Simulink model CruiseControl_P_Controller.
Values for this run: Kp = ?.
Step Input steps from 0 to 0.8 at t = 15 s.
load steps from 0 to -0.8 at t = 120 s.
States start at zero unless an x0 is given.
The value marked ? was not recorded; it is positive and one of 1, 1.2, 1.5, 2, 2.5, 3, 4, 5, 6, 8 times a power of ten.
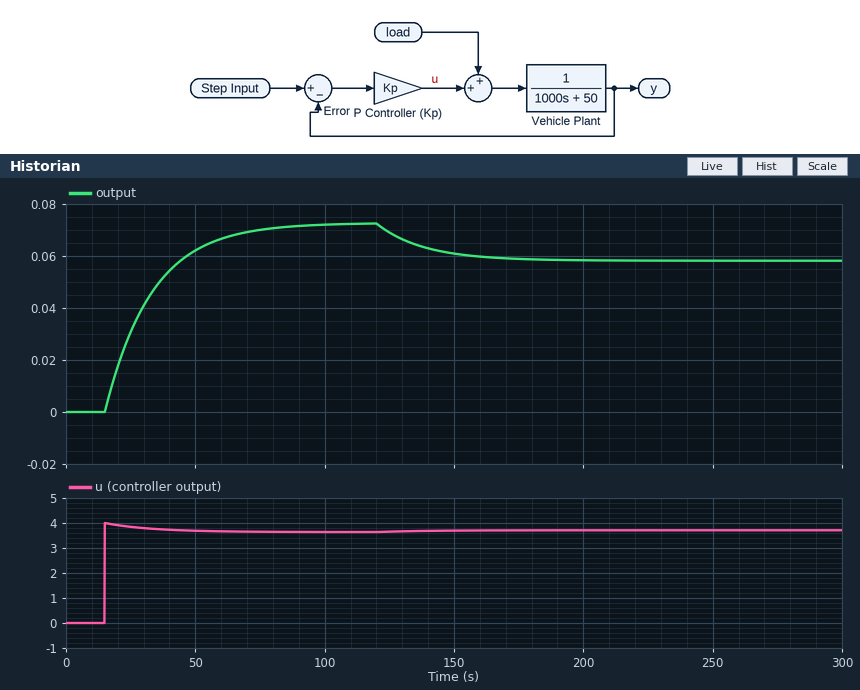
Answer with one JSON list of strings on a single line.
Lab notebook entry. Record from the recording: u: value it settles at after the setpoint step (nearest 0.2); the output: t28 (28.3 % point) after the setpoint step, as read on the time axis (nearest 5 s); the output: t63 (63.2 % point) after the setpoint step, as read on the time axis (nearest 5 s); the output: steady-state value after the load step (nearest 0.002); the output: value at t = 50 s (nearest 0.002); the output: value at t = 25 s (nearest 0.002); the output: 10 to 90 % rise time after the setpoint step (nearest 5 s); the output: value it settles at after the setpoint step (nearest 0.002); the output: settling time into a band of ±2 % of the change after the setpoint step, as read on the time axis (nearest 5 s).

["3.6", "20 s", "35 s", "0.058", "0.062", "0.030", "40 s", "0.072", "85 s"]
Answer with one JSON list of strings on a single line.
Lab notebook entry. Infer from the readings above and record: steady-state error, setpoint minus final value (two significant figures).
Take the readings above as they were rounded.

["0.73"]
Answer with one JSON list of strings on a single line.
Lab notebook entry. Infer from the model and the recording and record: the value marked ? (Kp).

["5"]
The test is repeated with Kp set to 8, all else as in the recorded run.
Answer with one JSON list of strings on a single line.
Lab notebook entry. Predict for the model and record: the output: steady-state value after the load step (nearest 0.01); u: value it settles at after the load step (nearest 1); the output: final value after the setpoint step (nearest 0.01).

["0.10", "6", "0.11"]
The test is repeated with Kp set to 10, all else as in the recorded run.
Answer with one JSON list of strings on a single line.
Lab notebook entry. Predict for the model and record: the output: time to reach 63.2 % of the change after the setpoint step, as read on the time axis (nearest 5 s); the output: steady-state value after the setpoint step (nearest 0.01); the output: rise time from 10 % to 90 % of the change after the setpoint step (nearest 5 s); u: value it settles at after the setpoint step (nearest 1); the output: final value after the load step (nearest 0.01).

["30 s", "0.13", "35 s", "7", "0.12"]
